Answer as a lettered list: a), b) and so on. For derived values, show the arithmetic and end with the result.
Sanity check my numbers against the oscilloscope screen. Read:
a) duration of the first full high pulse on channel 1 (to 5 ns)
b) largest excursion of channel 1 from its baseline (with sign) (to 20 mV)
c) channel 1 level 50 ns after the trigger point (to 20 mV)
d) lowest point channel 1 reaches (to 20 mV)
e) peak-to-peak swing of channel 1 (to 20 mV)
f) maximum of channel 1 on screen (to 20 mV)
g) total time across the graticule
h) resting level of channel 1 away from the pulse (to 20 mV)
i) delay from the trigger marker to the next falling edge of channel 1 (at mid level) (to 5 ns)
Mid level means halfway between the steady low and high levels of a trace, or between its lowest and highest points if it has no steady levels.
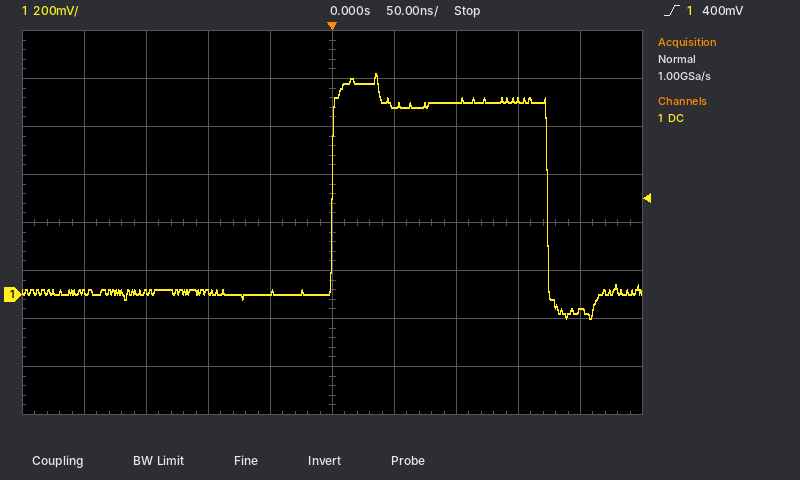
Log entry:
a) 175 ns
b) 920 mV − (0 mV) = +920 mV
c) 780 mV
d) -100 mV
e) 920 mV − (-100 mV) = 1.02 V
f) 920 mV
g) 500 ns
h) 0 mV
i) 175 ns
